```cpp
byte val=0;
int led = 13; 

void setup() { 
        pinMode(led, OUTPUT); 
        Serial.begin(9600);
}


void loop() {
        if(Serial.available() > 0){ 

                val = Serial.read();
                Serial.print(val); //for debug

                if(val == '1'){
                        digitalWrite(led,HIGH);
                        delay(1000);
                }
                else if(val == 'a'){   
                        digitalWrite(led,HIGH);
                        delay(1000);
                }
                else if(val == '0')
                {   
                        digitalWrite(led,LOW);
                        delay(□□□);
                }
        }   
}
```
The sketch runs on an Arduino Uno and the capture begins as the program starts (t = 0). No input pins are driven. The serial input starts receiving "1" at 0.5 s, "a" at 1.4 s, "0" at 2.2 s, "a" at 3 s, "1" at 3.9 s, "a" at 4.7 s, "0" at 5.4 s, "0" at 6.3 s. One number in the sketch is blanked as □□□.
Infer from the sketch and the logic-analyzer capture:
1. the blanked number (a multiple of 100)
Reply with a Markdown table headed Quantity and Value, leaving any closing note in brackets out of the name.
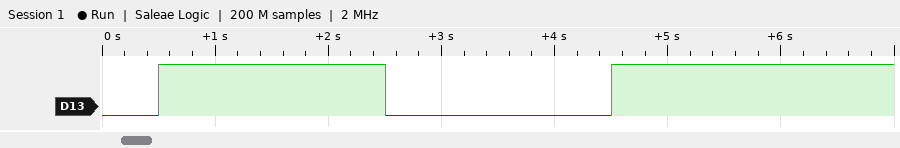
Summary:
| Quantity | Value |
|---|---|
| the blanked number | 2000 |
